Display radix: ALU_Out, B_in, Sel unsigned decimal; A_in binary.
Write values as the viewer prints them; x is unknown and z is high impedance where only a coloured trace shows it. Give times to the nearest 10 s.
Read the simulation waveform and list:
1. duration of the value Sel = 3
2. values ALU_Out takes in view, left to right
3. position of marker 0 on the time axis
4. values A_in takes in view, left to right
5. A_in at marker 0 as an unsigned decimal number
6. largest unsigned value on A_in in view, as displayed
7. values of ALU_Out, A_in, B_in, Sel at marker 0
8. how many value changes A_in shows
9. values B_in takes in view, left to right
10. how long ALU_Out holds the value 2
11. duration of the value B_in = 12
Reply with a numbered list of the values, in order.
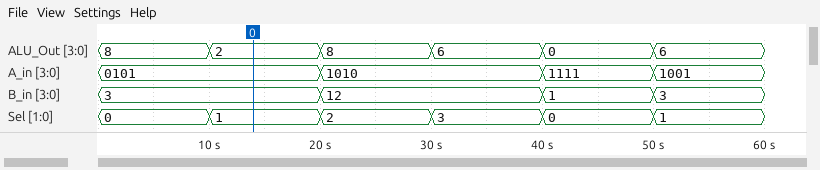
1. 10 s
2. 8, 2, 8, 6, 0, 6
3. 10 s
4. 0101, 1010, 1111, 1001
5. 5
6. 1111
7. ALU_Out=2, A_in=0101, B_in=3, Sel=1
8. 3
9. 3, 12, 1, 3
10. 10 s
11. 20 s
